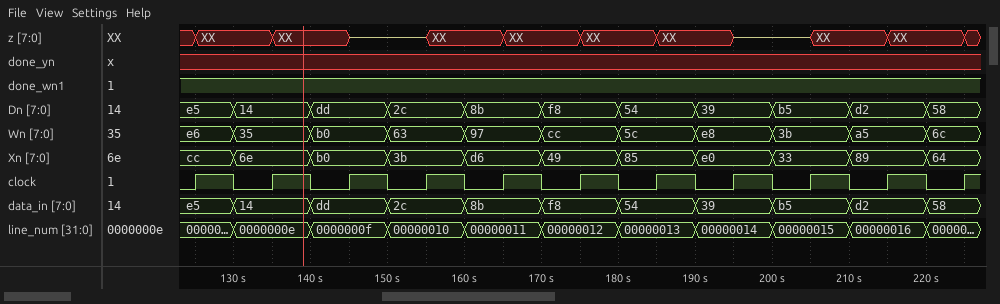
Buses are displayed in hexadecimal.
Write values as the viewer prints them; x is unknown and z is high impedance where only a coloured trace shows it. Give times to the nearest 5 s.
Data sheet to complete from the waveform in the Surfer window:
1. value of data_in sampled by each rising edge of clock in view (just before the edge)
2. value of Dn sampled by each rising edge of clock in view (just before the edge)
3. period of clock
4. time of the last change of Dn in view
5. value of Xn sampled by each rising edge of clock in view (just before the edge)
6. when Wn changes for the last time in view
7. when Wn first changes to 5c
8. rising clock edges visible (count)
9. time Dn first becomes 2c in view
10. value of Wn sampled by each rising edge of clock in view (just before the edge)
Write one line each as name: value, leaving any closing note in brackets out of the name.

value of data_in sampled by each rising edge of clock in view: e5, 14, dd, 2c, 8b, f8, 54, 39, b5, d2, 58
value of Dn sampled by each rising edge of clock in view: e5, 14, dd, 2c, 8b, f8, 54, 39, b5, d2, 58
period of clock: 10 s
time of the last change of Dn in view: 220 s
value of Xn sampled by each rising edge of clock in view: cc, 6e, b0, 3b, d6, 49, 85, e0, 33, 89, 64
when Wn changes for the last time in view: 220 s
when Wn first changes to 5c: 180 s
rising clock edges visible: 11
time Dn first becomes 2c in view: 150 s
value of Wn sampled by each rising edge of clock in view: e6, 35, b0, 63, 97, cc, 5c, e8, 3b, a5, 6c
